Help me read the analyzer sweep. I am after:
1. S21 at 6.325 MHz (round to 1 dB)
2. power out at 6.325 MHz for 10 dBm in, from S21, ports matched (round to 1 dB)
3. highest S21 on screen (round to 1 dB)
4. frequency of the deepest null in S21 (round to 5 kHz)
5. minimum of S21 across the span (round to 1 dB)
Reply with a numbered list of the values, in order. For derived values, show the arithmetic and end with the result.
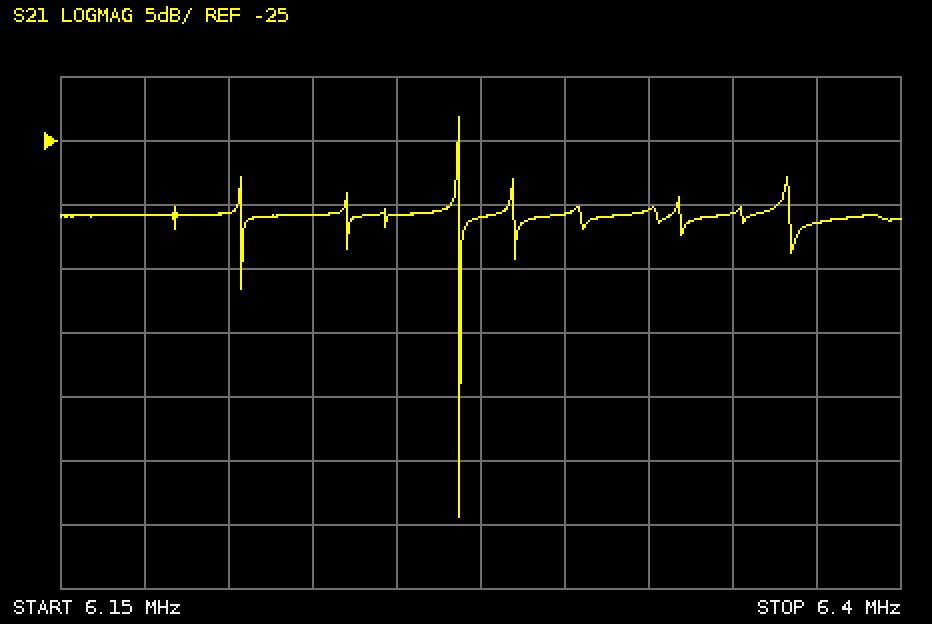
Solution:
1. -30 dB
2. 10 dBm + (-30 dB) = -20 dBm
3. -23 dB
4. 6.270 MHz
5. -54 dB
